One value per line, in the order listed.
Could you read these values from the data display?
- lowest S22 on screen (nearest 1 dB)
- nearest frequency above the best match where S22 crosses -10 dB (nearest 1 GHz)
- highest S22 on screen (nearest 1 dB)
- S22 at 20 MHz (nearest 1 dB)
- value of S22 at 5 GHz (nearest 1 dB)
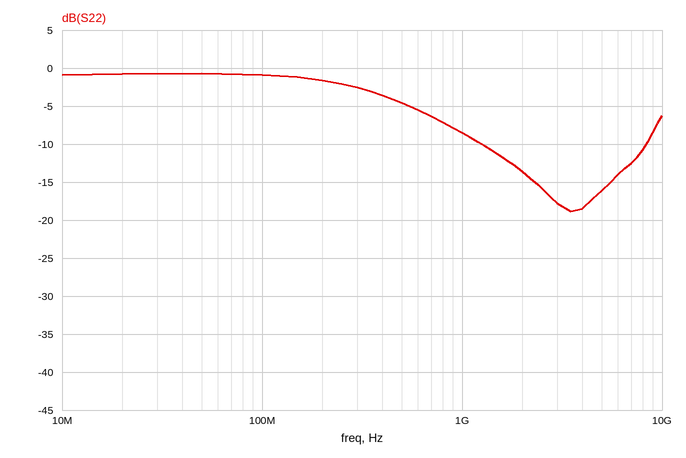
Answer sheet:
-19 dB
8 GHz
-1 dB
-1 dB
-16 dB
